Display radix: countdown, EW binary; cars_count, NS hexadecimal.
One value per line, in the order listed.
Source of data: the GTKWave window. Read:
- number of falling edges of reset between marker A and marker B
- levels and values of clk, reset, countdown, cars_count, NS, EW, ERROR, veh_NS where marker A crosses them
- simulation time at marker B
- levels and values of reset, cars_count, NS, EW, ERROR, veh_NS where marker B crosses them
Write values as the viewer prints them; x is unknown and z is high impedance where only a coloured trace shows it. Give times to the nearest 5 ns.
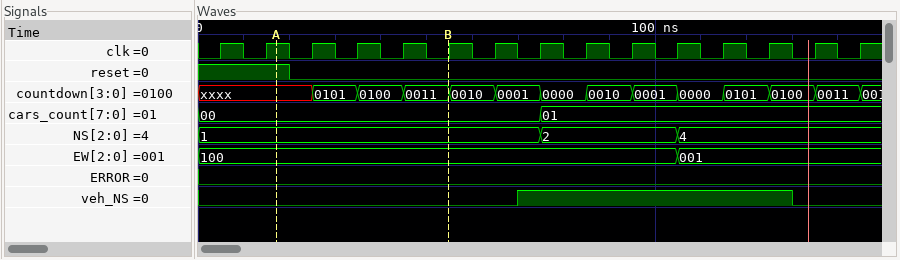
1
clk=1, reset=1, countdown=xxxx, cars_count=00, NS=1, EW=100, ERROR=0, veh_NS=0
55 ns
reset=0, cars_count=00, NS=1, EW=100, ERROR=0, veh_NS=0
